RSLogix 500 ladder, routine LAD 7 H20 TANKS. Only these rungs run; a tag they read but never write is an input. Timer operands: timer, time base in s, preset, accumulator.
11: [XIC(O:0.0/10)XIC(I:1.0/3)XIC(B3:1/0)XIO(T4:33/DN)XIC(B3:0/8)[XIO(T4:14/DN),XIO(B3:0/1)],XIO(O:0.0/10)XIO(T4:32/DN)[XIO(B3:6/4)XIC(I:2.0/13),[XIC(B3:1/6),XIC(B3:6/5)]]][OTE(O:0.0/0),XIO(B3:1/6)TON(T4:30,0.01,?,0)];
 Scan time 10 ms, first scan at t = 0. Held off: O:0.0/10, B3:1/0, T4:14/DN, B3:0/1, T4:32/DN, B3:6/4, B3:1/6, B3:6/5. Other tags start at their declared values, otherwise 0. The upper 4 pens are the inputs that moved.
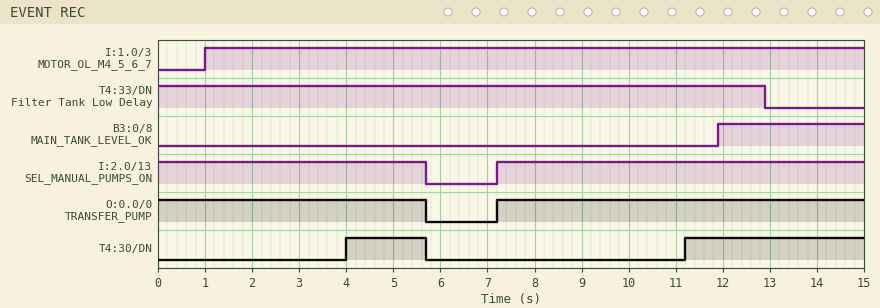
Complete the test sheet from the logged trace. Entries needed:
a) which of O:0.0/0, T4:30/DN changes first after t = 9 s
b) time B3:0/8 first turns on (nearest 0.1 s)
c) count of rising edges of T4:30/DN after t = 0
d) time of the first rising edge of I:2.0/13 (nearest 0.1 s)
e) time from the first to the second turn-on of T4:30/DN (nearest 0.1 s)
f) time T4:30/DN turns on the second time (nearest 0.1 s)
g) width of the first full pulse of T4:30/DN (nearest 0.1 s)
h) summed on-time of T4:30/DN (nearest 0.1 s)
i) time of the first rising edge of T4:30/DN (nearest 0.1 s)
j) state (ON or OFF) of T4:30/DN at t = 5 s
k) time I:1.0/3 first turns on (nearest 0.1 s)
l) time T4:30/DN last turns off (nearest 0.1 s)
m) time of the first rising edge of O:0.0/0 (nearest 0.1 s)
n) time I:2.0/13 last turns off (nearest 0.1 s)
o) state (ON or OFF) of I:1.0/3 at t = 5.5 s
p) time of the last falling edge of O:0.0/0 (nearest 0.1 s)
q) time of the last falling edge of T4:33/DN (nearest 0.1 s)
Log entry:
T4:30/DN
11.9 s
2
7.2 s
7.2 s
11.2 s
1.7 s
5.5 s
4.0 s
ON
1.0 s
5.7 s
7.2 s
5.7 s
ON
5.7 s
12.9 s
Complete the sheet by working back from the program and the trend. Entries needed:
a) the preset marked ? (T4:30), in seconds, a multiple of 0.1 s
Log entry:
4.0 s
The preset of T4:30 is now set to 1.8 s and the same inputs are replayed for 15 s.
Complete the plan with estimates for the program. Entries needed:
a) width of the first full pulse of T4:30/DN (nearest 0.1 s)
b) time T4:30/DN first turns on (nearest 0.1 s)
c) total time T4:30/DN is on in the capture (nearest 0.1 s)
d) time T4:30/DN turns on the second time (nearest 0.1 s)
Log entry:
3.9 s
1.8 s
9.9 s
9.0 s
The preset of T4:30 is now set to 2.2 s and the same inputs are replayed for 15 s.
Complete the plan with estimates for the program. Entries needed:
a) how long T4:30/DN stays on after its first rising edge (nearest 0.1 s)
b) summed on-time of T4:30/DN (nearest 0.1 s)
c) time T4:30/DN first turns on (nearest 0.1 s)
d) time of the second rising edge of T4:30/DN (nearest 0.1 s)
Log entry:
3.5 s
9.1 s
2.2 s
9.4 s
